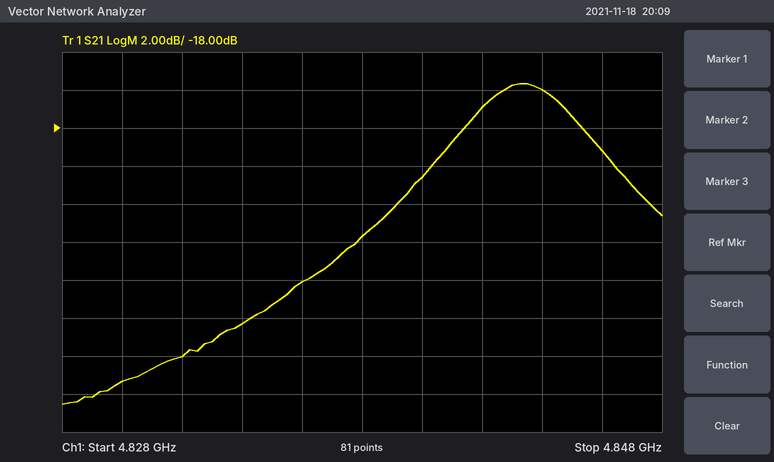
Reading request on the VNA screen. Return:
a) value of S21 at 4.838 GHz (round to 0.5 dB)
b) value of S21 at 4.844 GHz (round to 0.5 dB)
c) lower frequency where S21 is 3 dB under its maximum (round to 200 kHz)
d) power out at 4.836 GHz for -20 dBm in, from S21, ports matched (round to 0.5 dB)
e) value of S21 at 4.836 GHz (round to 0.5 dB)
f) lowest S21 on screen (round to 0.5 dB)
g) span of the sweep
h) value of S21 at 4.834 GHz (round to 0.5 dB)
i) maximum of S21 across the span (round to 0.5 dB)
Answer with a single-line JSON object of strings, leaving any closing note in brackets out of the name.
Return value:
{"value of S21 at 4.838 GHz": "-23.5 dB", "value of S21 at 4.844 GHz": "-16.0 dB", "lower frequency where S21 is 3 dB under its maximum": "4.8410 GHz", "power out at 4.836 GHz for -20 dBm in, from S21, ports matched": "-46.0 dBm", "value of S21 at 4.836 GHz": "-26.0 dB", "lowest S21 on screen": "-32.5 dB", "span of the sweep": "20 MHz", "value of S21 at 4.834 GHz": "-28.5 dB", "maximum of S21 across the span": "-15.5 dB"}
